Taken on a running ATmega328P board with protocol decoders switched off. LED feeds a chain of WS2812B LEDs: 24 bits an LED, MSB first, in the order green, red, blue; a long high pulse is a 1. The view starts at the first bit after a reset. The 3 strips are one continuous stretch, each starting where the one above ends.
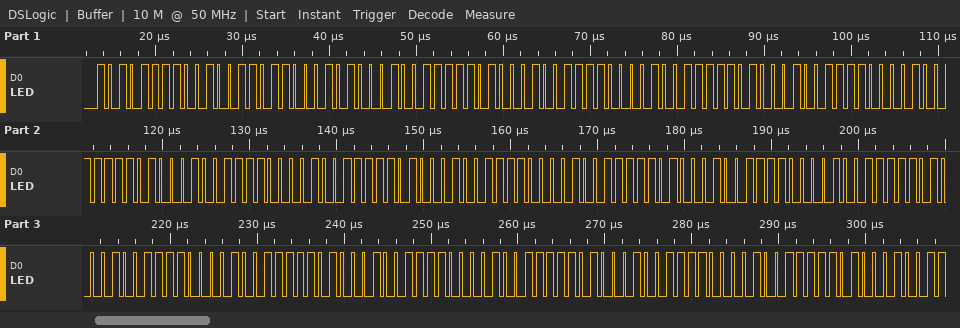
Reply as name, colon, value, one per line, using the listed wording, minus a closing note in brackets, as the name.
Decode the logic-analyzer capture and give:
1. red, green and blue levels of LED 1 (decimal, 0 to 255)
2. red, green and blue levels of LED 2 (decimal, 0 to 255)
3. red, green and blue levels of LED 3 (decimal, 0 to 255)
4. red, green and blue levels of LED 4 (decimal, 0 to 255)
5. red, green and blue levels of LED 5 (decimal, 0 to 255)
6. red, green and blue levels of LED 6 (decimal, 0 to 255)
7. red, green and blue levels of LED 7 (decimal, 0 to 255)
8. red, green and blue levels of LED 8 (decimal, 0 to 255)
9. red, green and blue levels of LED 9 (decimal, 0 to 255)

red, green and blue levels of LED 1: 38, 175, 197
red, green and blue levels of LED 2: 232, 19, 158
red, green and blue levels of LED 3: 232, 19, 158
red, green and blue levels of LED 4: 232, 19, 158
red, green and blue levels of LED 5: 232, 19, 158
red, green and blue levels of LED 6: 232, 19, 158
red, green and blue levels of LED 7: 232, 19, 158
red, green and blue levels of LED 8: 232, 19, 158
red, green and blue levels of LED 9: 232, 19, 158
